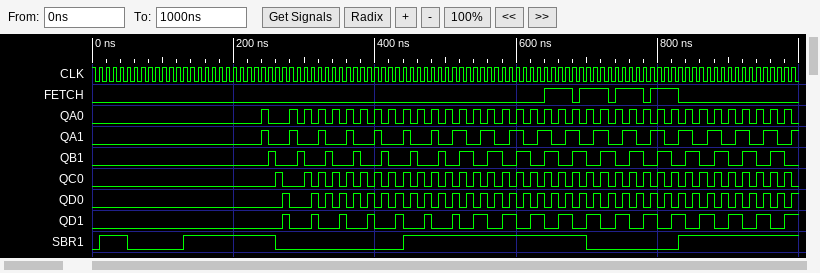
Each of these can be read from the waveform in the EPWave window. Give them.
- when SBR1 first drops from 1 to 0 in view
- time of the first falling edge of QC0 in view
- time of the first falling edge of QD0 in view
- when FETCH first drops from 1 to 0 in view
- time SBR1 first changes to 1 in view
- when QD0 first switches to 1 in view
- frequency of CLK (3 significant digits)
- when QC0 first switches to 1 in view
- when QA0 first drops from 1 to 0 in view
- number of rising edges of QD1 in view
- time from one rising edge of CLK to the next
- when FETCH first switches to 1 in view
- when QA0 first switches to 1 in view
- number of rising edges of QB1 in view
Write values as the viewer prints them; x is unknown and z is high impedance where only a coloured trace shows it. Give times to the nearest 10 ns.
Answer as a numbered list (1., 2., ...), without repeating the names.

1. 50 ns
2. 270 ns
3. 280 ns
4. 680 ns
5. 10 ns
6. 270 ns
7. 100 MHz
8. 260 ns
9. 250 ns
10. 19
11. 10 ns
12. 640 ns
13. 240 ns
14. 19
